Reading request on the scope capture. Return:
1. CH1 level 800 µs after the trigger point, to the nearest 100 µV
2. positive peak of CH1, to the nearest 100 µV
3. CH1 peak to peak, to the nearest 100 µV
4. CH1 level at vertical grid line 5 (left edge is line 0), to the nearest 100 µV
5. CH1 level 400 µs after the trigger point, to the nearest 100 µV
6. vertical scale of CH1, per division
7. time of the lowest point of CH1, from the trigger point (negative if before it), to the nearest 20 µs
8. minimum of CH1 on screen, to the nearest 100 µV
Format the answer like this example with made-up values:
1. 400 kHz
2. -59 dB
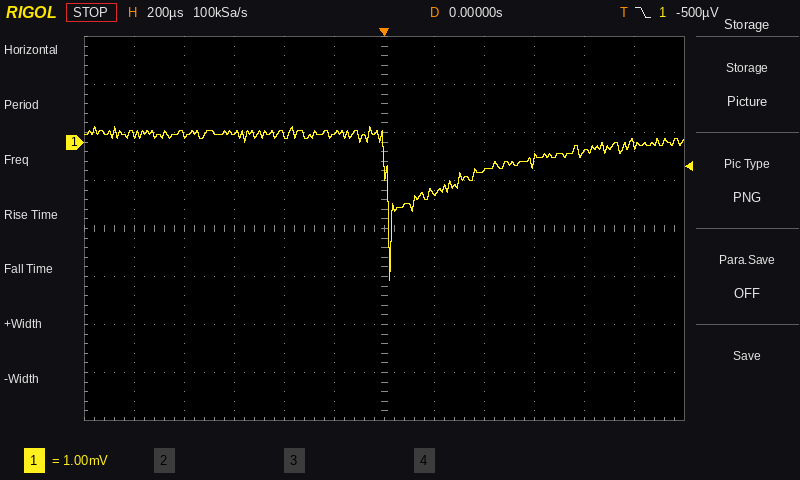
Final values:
1. -200 µV
2. 300 µV
3. 3.2 mV
4. 200 µV
5. -600 µV
6. 1 mV
7. +20 µs
8. -2.9 mV
